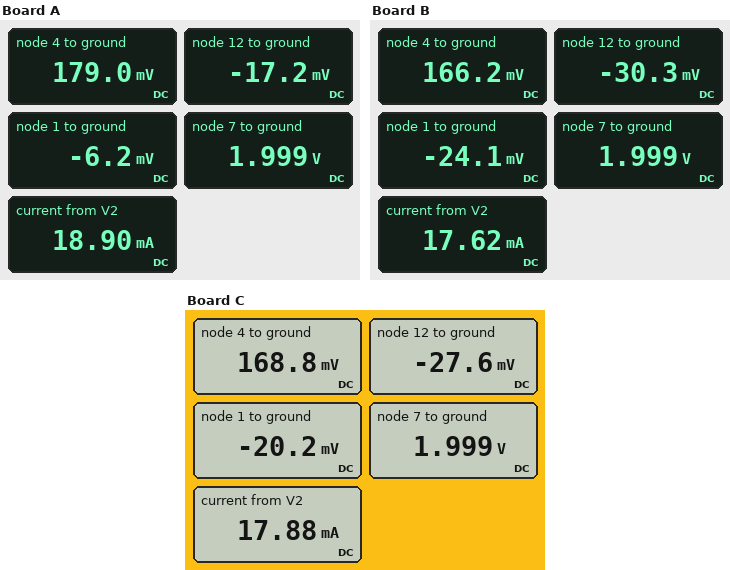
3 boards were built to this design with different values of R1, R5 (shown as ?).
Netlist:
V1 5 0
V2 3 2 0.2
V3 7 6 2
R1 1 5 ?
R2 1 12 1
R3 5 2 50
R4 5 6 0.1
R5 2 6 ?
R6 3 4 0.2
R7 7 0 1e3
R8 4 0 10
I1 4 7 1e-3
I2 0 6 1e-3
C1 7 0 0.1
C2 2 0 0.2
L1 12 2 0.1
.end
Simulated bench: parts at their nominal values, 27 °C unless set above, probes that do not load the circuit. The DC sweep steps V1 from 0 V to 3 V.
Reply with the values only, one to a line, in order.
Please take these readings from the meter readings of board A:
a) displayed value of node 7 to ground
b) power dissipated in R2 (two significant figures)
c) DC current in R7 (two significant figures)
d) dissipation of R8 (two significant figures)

1.999 V
120 µW
2.0 mA
3.2 mW
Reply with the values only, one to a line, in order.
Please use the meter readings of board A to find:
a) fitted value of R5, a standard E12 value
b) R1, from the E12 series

2.2 Ω
0.56 Ω
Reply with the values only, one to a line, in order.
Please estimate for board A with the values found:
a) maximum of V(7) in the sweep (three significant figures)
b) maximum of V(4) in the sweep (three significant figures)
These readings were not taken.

4.99 V
2.88 V
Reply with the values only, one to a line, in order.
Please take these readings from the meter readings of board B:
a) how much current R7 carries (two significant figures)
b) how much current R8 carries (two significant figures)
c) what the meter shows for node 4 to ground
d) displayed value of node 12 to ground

2.0 mA
17 mA
166.2 mV
-30.3 mV
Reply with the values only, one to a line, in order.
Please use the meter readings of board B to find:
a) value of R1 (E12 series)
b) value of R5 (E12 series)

3.9 Ω
2.7 Ω
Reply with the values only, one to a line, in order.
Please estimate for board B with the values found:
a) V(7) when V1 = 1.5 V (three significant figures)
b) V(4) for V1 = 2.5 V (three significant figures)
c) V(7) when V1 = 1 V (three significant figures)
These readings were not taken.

3.49 V
2.26 V
2.99 V
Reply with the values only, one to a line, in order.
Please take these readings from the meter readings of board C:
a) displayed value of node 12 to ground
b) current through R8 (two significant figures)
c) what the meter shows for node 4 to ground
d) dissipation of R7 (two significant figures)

-27.6 mV
17 mA
168.8 mV
4.0 mW
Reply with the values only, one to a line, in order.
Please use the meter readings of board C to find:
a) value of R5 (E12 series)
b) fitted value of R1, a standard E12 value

2.7 Ω
2.7 Ω
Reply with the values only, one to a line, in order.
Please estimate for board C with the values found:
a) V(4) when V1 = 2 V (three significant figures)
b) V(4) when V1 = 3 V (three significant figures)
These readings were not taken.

1.87 V
2.72 V
